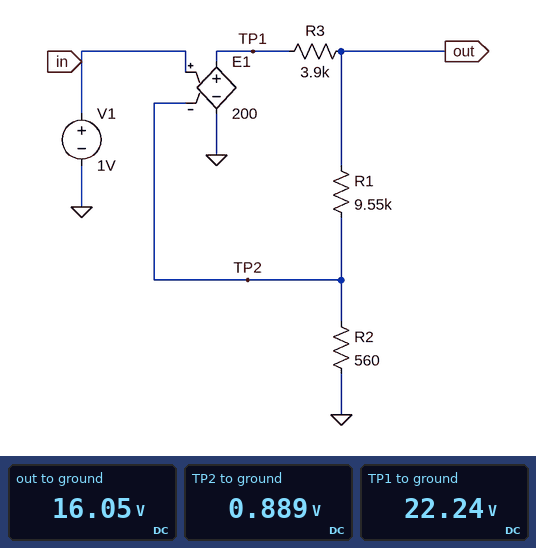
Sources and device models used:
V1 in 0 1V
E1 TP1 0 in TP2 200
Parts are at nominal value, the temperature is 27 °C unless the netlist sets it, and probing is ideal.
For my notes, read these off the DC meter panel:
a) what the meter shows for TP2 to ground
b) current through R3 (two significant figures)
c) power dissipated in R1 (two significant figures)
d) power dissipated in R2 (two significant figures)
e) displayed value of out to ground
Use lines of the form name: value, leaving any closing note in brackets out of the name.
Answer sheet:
what the meter shows for TP2 to ground: 0.889 V
current through R3: 1.6 mA
power dissipated in R1: 24 mW
power dissipated in R2: 1.4 mW
displayed value of out to ground: 16.05 V
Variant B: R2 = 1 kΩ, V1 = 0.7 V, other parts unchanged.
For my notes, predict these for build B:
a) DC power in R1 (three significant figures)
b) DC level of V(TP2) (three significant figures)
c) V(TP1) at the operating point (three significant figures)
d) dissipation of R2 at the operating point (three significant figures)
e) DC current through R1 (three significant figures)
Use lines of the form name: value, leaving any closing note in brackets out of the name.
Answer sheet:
DC power in R1: 4.07 mW
DC level of V(TP2): 653 mV
V(TP1) at the operating point: 9.43 V
dissipation of R2 at the operating point: 426 µW
DC current through R1: 653 µA
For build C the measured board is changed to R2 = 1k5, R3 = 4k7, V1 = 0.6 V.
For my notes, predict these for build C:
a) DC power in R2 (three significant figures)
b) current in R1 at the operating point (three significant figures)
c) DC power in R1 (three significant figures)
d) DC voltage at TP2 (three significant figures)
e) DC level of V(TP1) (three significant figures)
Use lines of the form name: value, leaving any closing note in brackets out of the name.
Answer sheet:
DC power in R2: 217 µW
current in R1 at the operating point: 380 µA
DC power in R1: 1.38 mW
DC voltage at TP2: 570 mV
DC level of V(TP1): 5.99 V
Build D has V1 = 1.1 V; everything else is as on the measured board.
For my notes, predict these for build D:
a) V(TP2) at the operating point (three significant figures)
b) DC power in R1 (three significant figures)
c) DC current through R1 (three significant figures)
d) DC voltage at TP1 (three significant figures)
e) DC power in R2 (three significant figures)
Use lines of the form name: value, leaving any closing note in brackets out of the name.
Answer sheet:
V(TP2) at the operating point: 978 mV
DC power in R1: 29.1 mW
DC current through R1: 1.75 mA
DC voltage at TP1: 24.5 V
DC power in R2: 1.71 mW
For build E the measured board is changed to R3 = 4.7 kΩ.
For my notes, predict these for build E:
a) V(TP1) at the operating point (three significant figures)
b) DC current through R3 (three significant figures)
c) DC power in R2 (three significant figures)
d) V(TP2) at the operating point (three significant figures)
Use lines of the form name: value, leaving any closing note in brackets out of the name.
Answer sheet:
V(TP1) at the operating point: 23.4 V
DC current through R3: 1.58 mA
DC power in R2: 1.39 mW
V(TP2) at the operating point: 883 mV
